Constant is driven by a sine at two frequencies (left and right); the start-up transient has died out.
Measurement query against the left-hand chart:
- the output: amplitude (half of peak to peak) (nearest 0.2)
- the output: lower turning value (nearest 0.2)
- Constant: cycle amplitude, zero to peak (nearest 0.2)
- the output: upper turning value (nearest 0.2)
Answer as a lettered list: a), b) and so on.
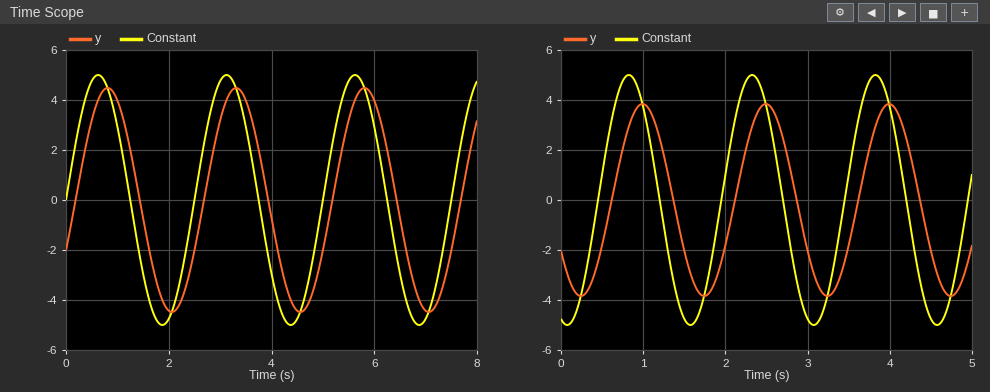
a) 4.4
b) -4.4
c) 5.0
d) 4.4
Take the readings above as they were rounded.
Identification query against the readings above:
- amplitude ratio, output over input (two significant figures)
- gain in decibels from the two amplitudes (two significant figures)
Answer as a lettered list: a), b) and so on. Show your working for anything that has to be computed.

a) 4.4 / 5 = 0.88
b) 20 log10(4.4 / 5) = -1.1 dB
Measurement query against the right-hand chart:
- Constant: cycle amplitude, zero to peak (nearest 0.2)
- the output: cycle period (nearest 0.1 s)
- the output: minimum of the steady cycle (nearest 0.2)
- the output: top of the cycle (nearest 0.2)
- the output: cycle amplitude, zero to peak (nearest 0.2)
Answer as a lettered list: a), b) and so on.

a) 5.0
b) 1.5 s
c) -3.8
d) 3.8
e) 3.8
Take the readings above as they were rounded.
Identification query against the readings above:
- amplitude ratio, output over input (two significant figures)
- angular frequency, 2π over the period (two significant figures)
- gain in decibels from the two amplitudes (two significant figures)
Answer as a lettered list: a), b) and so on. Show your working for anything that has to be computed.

a) 3.8 / 5 = 0.76
b) 2π / 1.5 = 4.2 rad/s
c) 20 log10(3.8 / 5) = -2.4 dB
